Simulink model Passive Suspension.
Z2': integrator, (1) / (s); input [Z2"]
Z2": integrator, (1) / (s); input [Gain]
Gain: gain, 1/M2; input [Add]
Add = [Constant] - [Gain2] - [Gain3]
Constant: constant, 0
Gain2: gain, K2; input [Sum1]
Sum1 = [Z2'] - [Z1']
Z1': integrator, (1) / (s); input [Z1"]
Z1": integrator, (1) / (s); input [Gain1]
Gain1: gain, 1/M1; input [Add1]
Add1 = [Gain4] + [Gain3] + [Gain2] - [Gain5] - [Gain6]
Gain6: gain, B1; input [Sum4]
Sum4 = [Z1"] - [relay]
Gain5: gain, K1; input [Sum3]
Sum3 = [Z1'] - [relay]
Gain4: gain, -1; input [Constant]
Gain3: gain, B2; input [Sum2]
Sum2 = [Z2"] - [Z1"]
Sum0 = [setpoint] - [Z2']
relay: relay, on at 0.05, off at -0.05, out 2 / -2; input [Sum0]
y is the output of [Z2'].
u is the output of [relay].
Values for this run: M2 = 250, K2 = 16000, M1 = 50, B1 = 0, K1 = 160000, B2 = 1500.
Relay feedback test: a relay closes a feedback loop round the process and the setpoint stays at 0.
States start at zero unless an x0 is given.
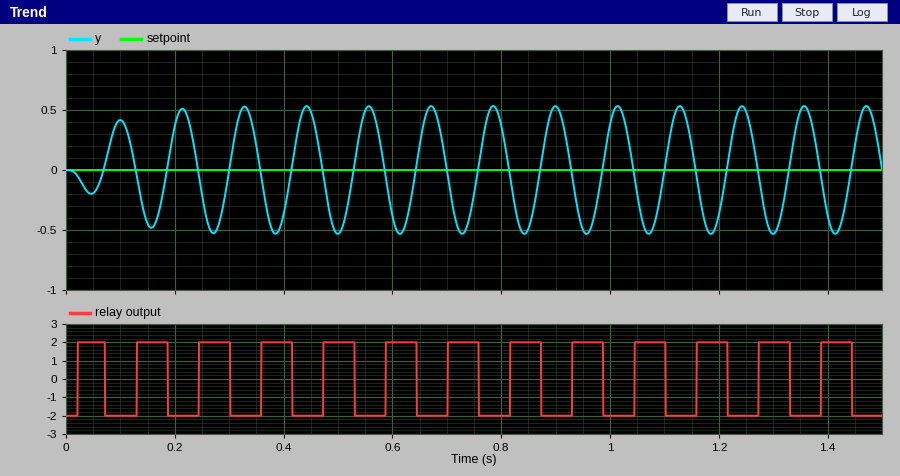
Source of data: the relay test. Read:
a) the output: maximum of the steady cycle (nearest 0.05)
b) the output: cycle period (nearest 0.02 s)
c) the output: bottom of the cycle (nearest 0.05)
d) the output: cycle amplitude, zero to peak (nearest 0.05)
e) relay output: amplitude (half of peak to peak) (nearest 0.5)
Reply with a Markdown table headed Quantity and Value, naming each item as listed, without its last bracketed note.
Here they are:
| Quantity | Value |
|---|---|
| the output: maximum of the steady cycle | 0.55 |
| the output: cycle period | 0.12 s |
| the output: bottom of the cycle | -0.55 |
| the output: cycle amplitude, zero to peak | 0.55 |
| relay output: amplitude (half of peak to peak) | 2.0 |
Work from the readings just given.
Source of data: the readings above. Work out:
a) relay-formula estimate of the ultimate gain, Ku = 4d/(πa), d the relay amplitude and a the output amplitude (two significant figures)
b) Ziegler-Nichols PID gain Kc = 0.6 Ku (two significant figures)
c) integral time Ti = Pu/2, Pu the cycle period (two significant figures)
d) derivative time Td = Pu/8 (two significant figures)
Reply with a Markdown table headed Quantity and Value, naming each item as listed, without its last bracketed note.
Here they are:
| Quantity | Value |
|---|---|
| relay-formula estimate of the ultimate gain, Ku = 4d/(πa), d the relay amplitude and a the output amplitude | 4.6 |
| Ziegler-Nichols PID gain Kc = 0.6 Ku | 2.8 |
| integral time Ti = Pu/2, Pu the cycle period | 0.060 s |
| derivative time Td = Pu/8 | 0.015 s |
